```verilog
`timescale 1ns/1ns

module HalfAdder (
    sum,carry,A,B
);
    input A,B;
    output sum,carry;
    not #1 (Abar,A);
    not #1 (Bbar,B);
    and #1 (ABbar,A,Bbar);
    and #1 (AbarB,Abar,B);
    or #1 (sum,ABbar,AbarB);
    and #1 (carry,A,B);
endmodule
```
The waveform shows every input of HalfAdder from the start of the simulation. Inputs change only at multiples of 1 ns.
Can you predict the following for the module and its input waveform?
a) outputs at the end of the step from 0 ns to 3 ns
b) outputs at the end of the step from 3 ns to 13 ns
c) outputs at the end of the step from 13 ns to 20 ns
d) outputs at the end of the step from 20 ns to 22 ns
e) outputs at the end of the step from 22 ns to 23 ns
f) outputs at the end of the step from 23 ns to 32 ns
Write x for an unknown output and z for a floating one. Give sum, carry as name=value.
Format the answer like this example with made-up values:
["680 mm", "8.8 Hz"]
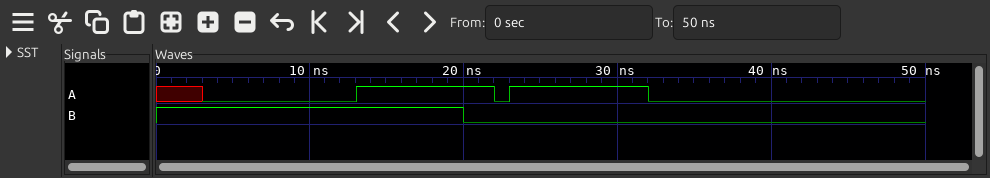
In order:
["sum=x, carry=x", "sum=1, carry=0", "sum=0, carry=1", "sum=0, carry=0", "sum=0, carry=0", "sum=1, carry=0"]
